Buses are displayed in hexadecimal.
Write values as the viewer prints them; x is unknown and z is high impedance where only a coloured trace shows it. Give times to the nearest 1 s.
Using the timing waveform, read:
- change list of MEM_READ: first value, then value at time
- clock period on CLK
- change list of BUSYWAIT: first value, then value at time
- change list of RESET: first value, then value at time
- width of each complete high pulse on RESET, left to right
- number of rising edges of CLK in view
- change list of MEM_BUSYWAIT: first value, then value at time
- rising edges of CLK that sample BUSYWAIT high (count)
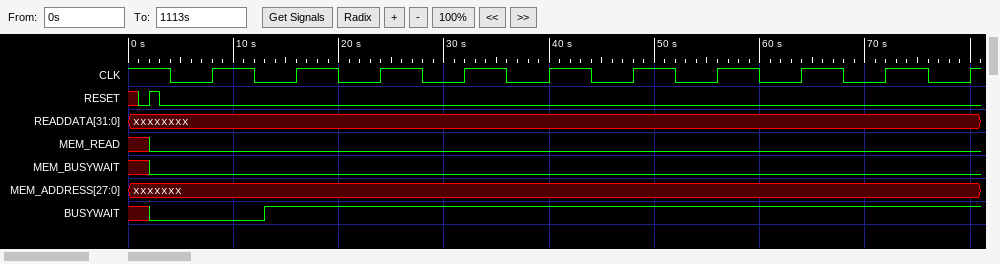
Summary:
x, 0 at 2 s
8 s
x, 0 at 2 s, 1 at 13 s
x, 0 at 1 s, 1 at 2 s, 0 at 3 s
1 s
10
x, 0 at 2 s
9
